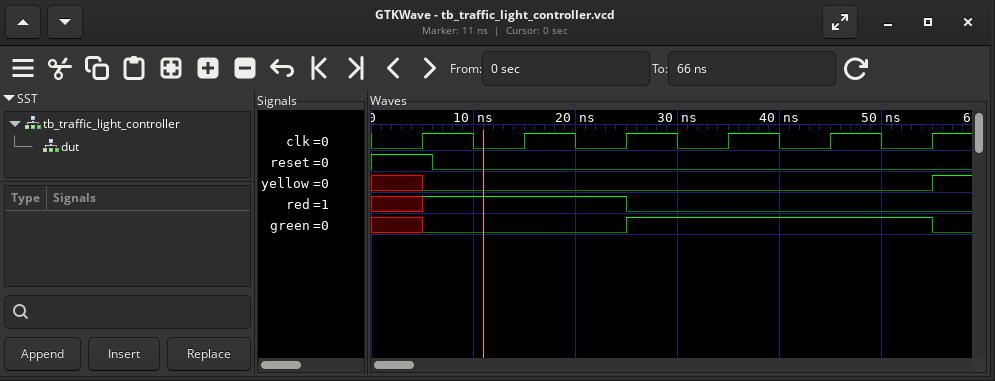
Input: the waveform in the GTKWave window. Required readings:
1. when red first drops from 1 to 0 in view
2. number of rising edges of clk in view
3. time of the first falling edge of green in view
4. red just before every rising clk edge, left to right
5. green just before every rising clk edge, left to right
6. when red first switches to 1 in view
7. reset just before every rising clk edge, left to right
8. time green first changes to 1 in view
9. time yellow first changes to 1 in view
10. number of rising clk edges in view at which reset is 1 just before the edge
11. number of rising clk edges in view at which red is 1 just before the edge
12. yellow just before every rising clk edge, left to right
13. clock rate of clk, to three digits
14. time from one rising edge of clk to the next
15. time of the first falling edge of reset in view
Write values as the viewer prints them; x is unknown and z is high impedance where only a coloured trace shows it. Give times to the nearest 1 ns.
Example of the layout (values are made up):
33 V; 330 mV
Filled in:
25 ns; 6; 55 ns; x 1 1 0 0 0; x 0 0 1 1 1; 5 ns; 1 0 0 0 0 0; 25 ns; 55 ns; 1; 2; x 0 0 0 0 0; 100 MHz; 10 ns; 6 ns
